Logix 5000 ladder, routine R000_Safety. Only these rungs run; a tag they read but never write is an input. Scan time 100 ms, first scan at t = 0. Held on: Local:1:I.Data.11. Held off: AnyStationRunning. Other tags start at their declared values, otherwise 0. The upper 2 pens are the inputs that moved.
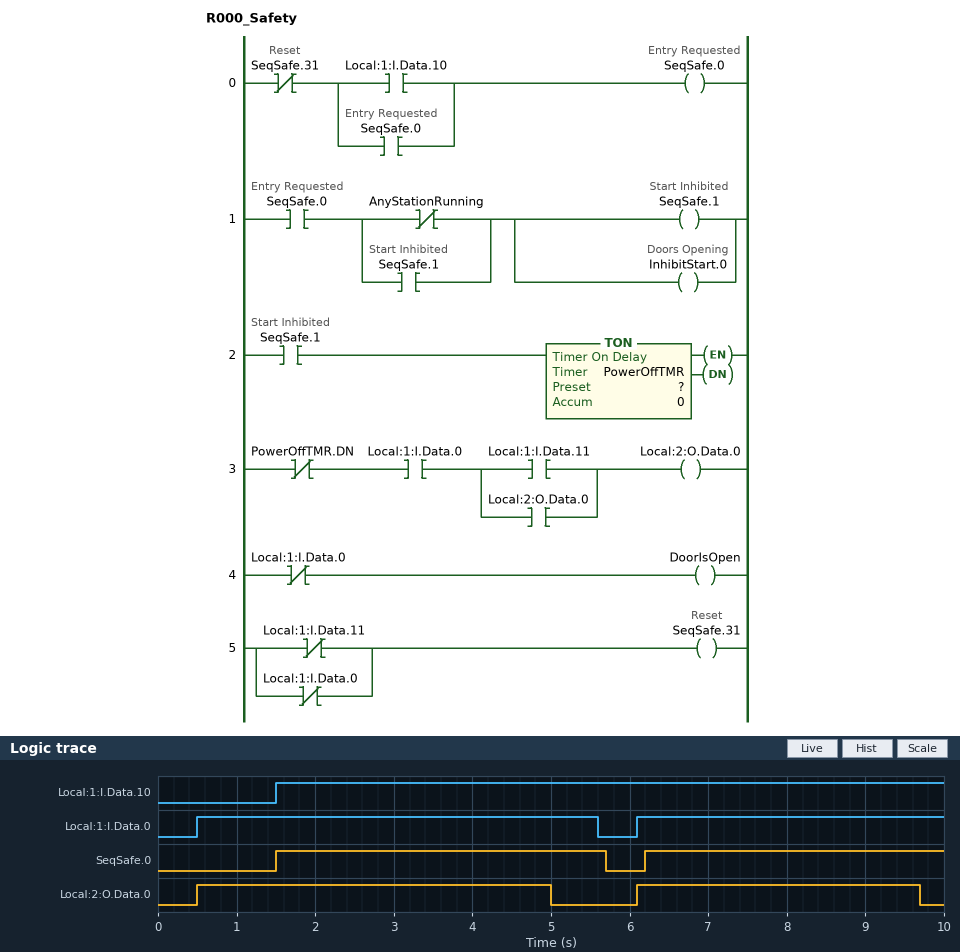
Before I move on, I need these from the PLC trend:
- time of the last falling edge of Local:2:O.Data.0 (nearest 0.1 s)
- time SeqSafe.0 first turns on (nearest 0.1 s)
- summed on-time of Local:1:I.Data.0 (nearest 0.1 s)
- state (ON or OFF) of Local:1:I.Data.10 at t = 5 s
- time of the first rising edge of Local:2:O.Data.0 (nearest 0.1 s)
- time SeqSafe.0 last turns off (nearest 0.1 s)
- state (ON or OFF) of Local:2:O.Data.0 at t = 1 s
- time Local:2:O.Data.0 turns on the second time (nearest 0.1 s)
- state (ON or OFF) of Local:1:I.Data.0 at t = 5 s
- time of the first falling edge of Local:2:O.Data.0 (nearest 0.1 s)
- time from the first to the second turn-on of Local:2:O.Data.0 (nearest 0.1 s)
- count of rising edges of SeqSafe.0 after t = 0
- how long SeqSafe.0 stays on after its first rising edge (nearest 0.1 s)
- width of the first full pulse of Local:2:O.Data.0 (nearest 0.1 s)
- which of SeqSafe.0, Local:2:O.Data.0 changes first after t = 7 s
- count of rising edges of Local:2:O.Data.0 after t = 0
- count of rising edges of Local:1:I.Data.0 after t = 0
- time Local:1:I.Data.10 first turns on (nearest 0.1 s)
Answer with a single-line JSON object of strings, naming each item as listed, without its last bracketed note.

{"time of the last falling edge of Local:2:O.Data.0": "9.7 s", "time SeqSafe.0 first turns on": "1.5 s", "summed on-time of Local:1:I.Data.0": "9.0 s", "state (ON or OFF) of Local:1:I.Data.10 at t = 5 s": "ON", "time of the first rising edge of Local:2:O.Data.0": "0.5 s", "time SeqSafe.0 last turns off": "5.7 s", "state (ON or OFF) of Local:2:O.Data.0 at t = 1 s": "ON", "time Local:2:O.Data.0 turns on the second time": "6.1 s", "state (ON or OFF) of Local:1:I.Data.0 at t = 5 s": "ON", "time of the first falling edge of Local:2:O.Data.0": "5.0 s", "time from the first to the second turn-on of Local:2:O.Data.0": "5.6 s", "count of rising edges of SeqSafe.0 after t = 0": "2", "how long SeqSafe.0 stays on after its first rising edge": "4.2 s", "width of the first full pulse of Local:2:O.Data.0": "4.5 s", "which of SeqSafe.0, Local:2:O.Data.0 changes first after t = 7 s": "Local:2:O.Data.0", "count of rising edges of Local:2:O.Data.0 after t = 0": "2", "count of rising edges of Local:1:I.Data.0 after t = 0": "2", "time Local:1:I.Data.10 first turns on": "1.5 s"}
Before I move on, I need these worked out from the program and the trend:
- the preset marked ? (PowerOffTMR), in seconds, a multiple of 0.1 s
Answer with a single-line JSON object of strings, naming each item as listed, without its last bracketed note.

{"the preset marked ? (PowerOffTMR), in seconds, a multiple of 0.1 s": "3.5 s"}
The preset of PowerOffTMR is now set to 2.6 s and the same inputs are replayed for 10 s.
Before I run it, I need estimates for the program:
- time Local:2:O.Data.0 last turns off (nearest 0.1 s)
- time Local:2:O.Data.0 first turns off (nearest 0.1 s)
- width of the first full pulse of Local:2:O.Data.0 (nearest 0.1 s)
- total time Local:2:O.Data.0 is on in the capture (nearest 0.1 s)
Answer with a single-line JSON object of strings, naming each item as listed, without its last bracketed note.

{"time Local:2:O.Data.0 last turns off": "8.8 s", "time Local:2:O.Data.0 first turns off": "4.1 s", "width of the first full pulse of Local:2:O.Data.0": "3.6 s", "total time Local:2:O.Data.0 is on in the capture": "6.3 s"}
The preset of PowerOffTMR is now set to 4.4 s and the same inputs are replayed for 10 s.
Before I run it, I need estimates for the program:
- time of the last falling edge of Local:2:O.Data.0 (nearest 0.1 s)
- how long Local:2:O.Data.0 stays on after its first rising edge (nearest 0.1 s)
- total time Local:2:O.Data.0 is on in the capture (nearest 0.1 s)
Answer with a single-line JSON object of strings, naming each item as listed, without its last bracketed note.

{"time of the last falling edge of Local:2:O.Data.0": "5.6 s", "how long Local:2:O.Data.0 stays on after its first rising edge": "5.1 s", "total time Local:2:O.Data.0 is on in the capture": "9.0 s"}
